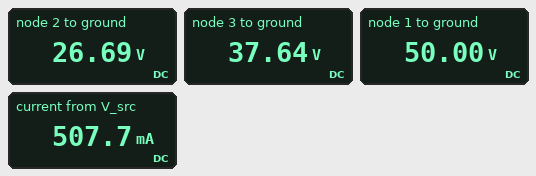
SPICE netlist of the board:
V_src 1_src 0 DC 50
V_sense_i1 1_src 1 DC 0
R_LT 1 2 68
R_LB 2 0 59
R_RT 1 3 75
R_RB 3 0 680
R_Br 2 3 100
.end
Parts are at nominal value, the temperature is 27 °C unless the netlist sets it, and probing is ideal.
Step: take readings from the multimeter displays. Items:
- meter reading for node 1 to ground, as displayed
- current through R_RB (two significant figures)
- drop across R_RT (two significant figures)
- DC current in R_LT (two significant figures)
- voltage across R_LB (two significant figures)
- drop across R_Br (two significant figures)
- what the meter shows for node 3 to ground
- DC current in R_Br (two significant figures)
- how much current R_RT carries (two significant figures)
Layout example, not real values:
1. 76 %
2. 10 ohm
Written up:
1. 50.00 V
2. 55 mA
3. 12 V
4. 340 mA
5. 27 V
6. 11 V
7. 37.64 V
8. 110 mA
9. 160 mA
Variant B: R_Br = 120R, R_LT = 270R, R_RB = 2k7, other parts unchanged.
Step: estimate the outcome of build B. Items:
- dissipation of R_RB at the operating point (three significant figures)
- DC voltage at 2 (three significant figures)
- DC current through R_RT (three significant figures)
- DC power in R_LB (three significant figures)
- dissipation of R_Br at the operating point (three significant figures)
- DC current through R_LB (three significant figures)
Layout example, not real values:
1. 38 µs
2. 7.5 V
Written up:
1. 498 mW
2. 16.9 V
3. 178 mA
4. 4.86 W
5. 3.24 W
6. 287 mA
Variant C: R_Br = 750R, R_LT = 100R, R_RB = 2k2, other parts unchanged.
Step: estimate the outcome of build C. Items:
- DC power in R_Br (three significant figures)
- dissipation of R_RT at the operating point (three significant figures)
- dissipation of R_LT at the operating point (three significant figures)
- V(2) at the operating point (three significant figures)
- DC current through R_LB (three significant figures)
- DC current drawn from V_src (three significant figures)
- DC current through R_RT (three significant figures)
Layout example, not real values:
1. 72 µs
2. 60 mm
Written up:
1. 901 mW
2. 231 mW
3. 9.10 W
4. 19.8 V
5. 336 mA
6. 357 mA
7. 55.5 mA
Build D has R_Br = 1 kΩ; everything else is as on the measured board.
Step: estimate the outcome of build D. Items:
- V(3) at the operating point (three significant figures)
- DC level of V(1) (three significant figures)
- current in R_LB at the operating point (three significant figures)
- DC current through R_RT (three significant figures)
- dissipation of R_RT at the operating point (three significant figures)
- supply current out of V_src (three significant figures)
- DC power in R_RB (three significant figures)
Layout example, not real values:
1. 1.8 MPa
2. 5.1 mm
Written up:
1. 43.7 V
2. 50.0 V
3. 404 mA
4. 84.1 mA
5. 530 mW
6. 469 mA
7. 2.81 W
